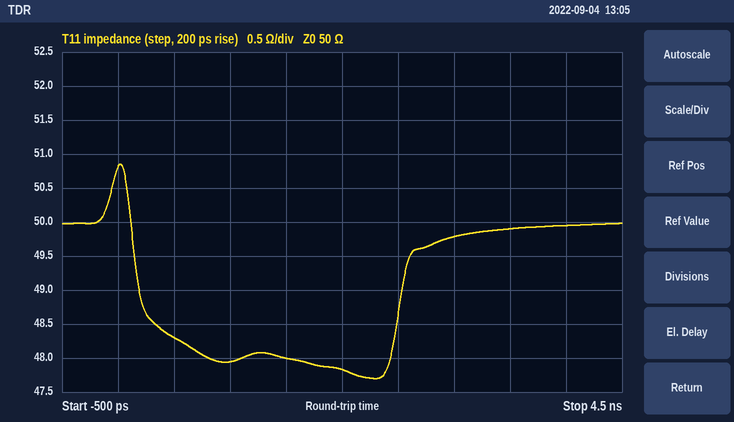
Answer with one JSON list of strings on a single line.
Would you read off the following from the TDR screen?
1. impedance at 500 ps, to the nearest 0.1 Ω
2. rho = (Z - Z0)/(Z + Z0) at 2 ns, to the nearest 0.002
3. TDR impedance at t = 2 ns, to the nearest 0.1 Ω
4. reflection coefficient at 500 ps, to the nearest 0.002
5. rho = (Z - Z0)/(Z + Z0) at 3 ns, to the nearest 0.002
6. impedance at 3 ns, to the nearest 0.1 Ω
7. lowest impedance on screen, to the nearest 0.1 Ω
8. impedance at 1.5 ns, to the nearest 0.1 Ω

["48.3 Ω", "-0.022", "47.8 Ω", "-0.018", "-0.002", "49.8 Ω", "47.7 Ω", "48.0 Ω"]
